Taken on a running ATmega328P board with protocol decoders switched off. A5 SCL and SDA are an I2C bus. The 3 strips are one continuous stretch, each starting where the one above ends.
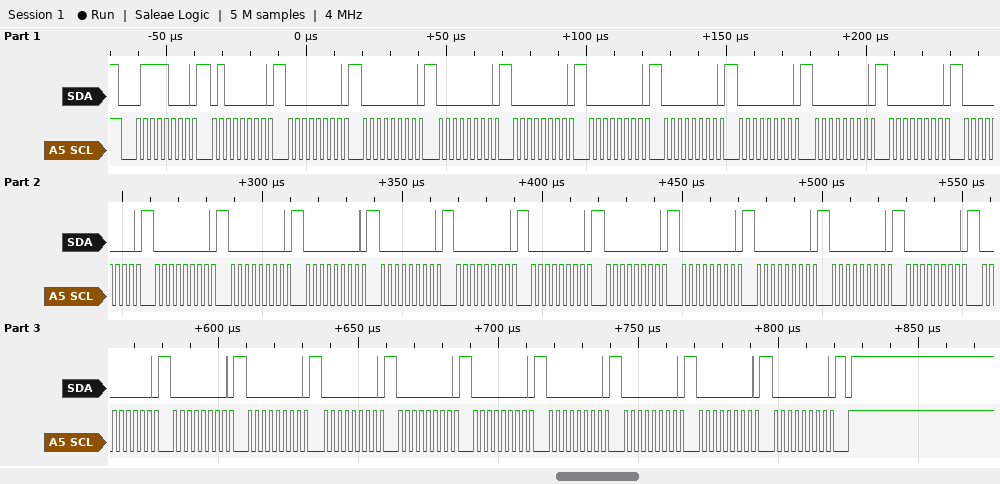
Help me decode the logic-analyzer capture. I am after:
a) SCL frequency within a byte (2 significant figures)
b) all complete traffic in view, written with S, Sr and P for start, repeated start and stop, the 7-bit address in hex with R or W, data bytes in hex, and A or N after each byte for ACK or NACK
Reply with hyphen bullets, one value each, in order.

- 400 kHz
- S 3CW A 40 A 00 A 00 A 00 A 00 A 00 A 00 A 00 A 00 A 00 A 00 A 00 A 00 A 00 A 00 A 00 A 00 A 00 A 00 A 00 A 00 A 00 A 00 A 00 A 00 A 00 A 00 A 00 A 00 A 00 A 00 A 00 A P
